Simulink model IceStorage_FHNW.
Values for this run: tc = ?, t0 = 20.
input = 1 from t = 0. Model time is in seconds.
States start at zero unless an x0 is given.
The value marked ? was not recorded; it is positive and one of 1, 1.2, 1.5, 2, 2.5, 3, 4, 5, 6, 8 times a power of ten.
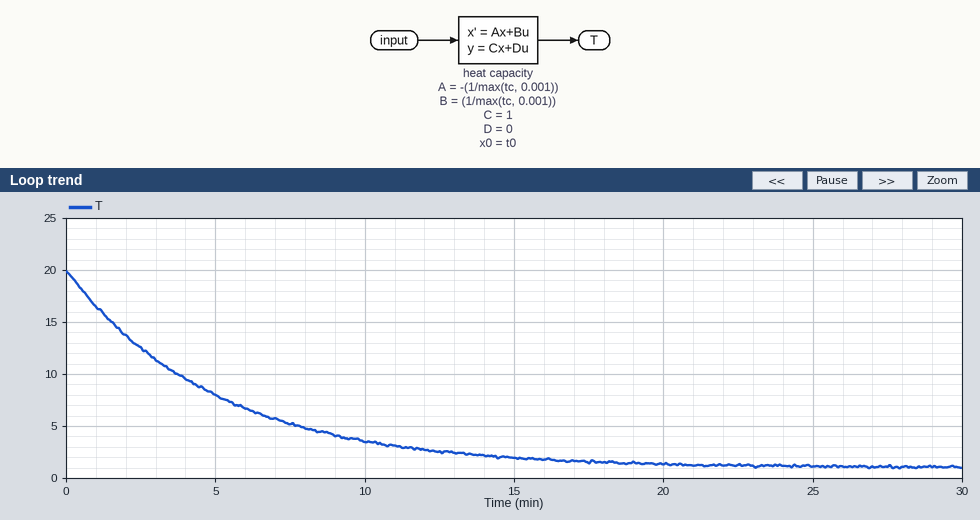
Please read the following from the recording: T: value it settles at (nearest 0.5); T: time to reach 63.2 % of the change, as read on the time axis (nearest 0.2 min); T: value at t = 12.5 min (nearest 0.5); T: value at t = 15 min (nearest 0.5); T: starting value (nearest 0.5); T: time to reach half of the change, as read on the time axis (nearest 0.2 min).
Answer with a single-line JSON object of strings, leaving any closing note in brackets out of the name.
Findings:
{"T: value it settles at": "1.0", "T: time to reach 63.2 % of the change, as read on the time axis": "5.0 min", "T: value at t = 12.5 min": "2.5", "T: value at t = 15 min": "2.0", "T: starting value": "20.0", "T: time to reach half of the change, as read on the time axis": "3.4 min"}
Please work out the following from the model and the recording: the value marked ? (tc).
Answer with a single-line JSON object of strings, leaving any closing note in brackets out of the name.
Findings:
{"the value marked ?": "300"}
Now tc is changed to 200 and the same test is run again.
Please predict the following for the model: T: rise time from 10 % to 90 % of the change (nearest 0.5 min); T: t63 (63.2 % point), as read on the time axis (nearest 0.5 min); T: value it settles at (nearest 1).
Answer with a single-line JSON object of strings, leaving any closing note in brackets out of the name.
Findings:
{"T: rise time from 10 % to 90 % of the change": "7.5 min", "T: t63 (63.2 % point), as read on the time axis": "3.5 min", "T: value it settles at": "1"}
